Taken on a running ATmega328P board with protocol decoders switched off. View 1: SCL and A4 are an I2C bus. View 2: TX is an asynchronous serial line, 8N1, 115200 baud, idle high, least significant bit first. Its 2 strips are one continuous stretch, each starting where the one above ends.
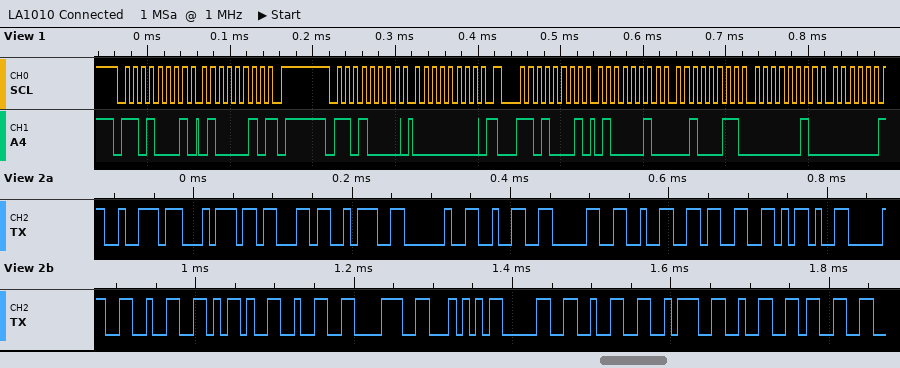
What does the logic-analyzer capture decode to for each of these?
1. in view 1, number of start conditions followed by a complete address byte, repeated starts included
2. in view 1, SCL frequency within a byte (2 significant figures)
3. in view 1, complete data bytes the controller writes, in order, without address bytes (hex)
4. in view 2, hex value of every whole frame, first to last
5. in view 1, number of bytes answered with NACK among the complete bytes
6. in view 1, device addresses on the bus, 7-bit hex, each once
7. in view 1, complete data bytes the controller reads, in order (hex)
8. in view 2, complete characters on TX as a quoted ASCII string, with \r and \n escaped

3
100 kHz
00
72 74 63 3A 20 32 30 32 33 2D 30 32 2D 32 38 54 30 32 3A 32 33
1
0x68
42 42 23 02
"rtc: 2023-02-28T02:23"
